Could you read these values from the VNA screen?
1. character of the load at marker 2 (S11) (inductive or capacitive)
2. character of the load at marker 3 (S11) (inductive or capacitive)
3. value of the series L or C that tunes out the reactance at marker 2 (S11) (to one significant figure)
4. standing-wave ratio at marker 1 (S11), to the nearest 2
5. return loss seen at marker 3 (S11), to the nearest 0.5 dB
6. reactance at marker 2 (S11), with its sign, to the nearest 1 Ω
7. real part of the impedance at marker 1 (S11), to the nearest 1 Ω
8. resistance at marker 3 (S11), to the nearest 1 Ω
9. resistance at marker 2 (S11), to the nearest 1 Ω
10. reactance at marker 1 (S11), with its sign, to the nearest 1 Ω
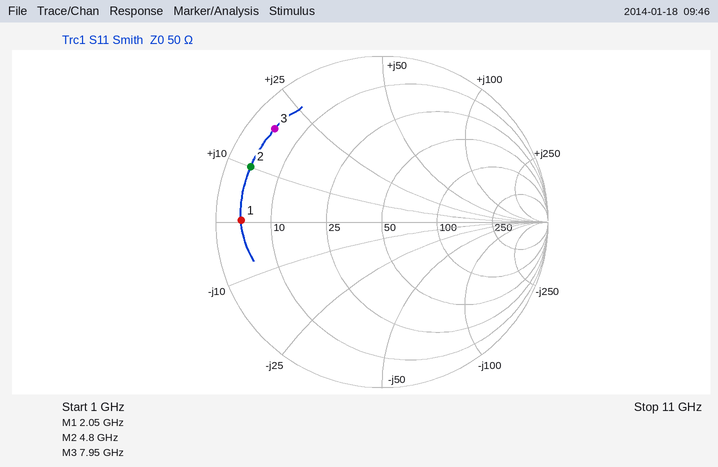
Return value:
inductive
inductive
3 pF
12
1.5 dB
+10 Ω
4 Ω
4 Ω
4 Ω
0 Ω
